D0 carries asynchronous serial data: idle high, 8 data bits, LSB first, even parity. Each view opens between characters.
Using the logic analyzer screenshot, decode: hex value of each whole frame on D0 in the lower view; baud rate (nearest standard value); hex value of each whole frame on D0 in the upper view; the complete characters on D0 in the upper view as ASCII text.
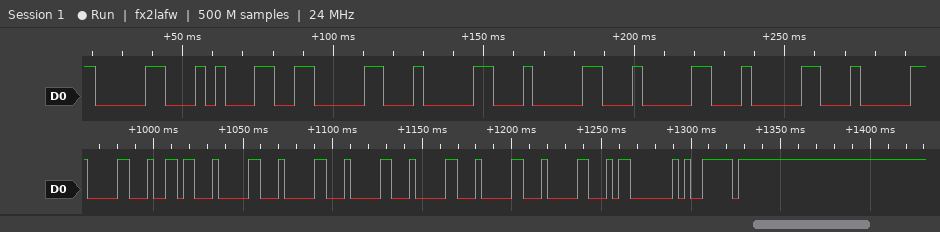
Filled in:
30, 36, 30, 30, 30, 30, 30, 30, 03, F9
300 baud
30, 31, 30, 30, 30, 30, 30
"0100000"
